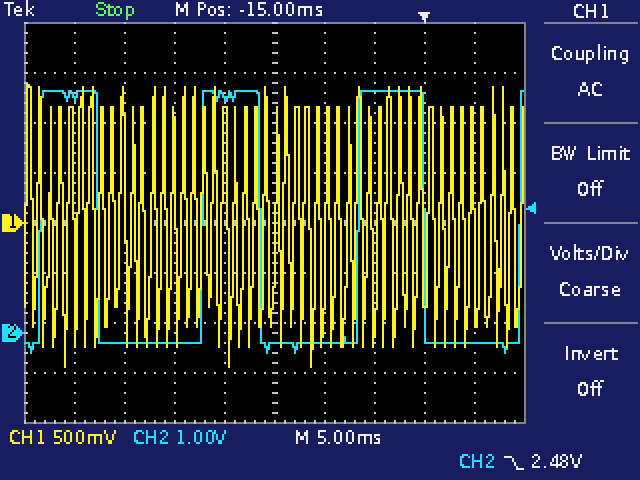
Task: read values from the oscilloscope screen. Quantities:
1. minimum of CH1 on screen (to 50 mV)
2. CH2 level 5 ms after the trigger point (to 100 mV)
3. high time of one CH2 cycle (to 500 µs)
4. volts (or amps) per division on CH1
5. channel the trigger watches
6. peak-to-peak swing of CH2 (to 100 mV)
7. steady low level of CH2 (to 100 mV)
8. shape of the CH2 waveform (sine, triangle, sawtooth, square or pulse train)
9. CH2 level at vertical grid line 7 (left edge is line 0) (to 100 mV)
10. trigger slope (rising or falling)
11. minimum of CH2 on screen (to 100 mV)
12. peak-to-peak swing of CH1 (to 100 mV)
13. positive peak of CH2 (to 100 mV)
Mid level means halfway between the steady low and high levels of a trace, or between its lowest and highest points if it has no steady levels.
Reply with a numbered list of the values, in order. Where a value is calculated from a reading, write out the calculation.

1. -1.45 V
2. -200 mV
3. 6.0 ms
4. 500 mV
5. CH2
6. 4.8 V − (-400 mV) = 5.2 V
7. -200 mV
8. pulse train
9. 4.8 V
10. falling
11. -400 mV
12. 2.80 V
13. 4.8 V
